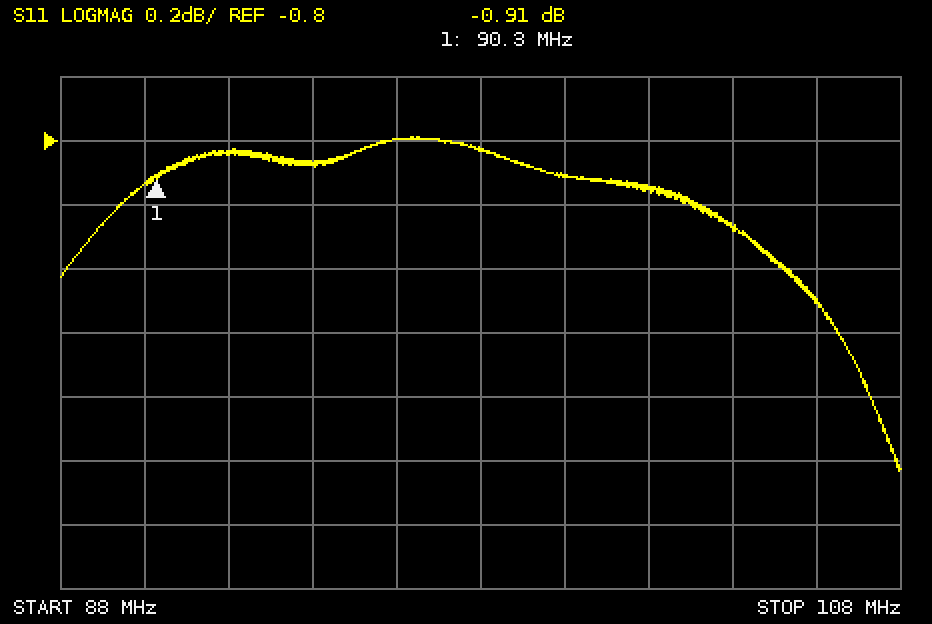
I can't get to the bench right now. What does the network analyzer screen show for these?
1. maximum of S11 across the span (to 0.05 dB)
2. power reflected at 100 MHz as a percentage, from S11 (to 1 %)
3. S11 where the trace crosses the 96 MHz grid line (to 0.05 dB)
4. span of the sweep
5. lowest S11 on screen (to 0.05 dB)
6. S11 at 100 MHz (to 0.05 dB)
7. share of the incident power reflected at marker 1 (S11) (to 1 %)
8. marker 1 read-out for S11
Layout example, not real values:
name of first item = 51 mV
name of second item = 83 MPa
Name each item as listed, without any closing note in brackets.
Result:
maximum of S11 across the span = -0.80 dB
power reflected at 100 MHz as a percentage, from S11 = 81 %
S11 where the trace crosses the 96 MHz grid line = -0.80 dB
span of the sweep = 20 MHz
lowest S11 on screen = -1.85 dB
S11 at 100 MHz = -0.90 dB
share of the incident power reflected at marker 1 (S11) = 81 %
marker 1 read-out for S11 = -0.91 dB
